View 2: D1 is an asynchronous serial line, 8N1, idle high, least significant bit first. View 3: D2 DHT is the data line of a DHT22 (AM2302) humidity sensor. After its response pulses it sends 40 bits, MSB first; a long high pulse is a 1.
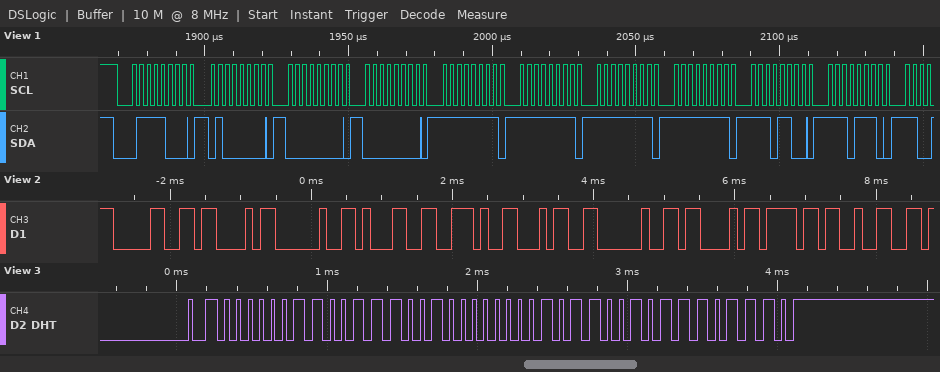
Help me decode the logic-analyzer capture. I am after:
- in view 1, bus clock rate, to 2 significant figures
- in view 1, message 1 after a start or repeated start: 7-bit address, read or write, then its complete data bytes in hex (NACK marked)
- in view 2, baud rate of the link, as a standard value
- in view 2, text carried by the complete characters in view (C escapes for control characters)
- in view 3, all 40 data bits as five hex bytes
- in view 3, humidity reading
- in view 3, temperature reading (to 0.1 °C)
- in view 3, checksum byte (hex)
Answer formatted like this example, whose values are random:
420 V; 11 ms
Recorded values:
400 kHz; 0x3C write: 40 00 00 FF FF FF FF EC EE; 9600 baud; "0C 1.4 Co2"; 03 39 00 B2 EE; 82.5 %; 17.8 °C; 0xEE
